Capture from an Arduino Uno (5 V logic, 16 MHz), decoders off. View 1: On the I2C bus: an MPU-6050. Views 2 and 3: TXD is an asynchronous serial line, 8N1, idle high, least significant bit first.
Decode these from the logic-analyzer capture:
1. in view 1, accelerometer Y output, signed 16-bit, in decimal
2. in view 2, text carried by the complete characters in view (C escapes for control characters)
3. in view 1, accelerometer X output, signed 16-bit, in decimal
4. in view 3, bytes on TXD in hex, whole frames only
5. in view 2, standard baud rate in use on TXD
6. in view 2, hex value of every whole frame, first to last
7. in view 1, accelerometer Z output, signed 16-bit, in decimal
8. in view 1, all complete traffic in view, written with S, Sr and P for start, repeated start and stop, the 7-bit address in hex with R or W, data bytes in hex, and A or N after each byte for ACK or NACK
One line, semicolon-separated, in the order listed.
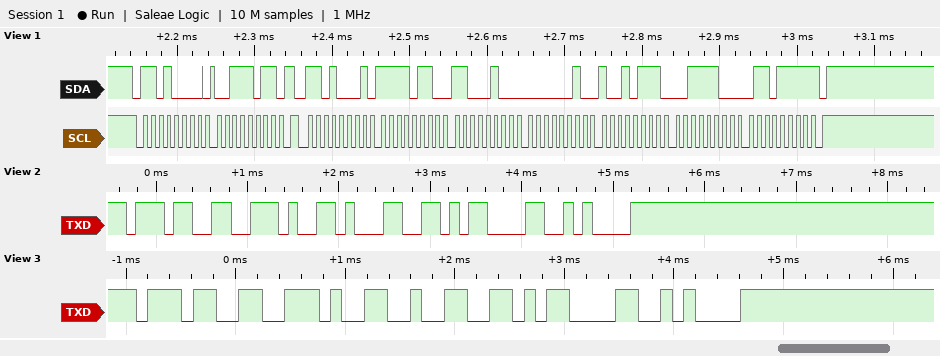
663; "7.1\r\n"; -2364; 37 2E 32 0D 0A; 9600 baud; 0x37 0x2E 0x31 0x0D 0x0A; 15471; S 68W A 3B A Sr 68R A F6 A C4 A 02 A 97 A 3C A 6F N P
